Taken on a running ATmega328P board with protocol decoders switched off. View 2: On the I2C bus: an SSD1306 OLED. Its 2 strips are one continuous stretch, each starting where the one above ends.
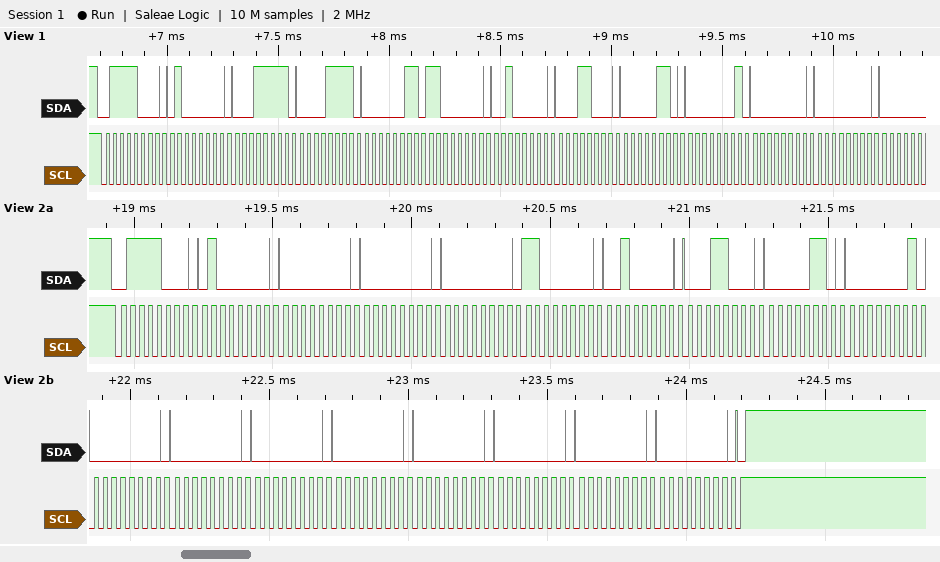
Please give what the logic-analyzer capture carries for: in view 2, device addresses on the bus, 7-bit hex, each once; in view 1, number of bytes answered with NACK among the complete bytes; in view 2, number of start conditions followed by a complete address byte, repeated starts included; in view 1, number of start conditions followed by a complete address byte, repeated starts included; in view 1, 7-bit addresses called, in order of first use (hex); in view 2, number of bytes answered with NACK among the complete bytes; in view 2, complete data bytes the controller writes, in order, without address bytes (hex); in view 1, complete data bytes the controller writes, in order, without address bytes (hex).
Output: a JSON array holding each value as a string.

["0x3C", "0", "1", "1", "0x3C", "0", "40 00 00 00 C0 20 18 06 01 00 00 00 00 00 00 00 00", "40 1F 0F 03 C0 20 18 06 01 00 00"]
